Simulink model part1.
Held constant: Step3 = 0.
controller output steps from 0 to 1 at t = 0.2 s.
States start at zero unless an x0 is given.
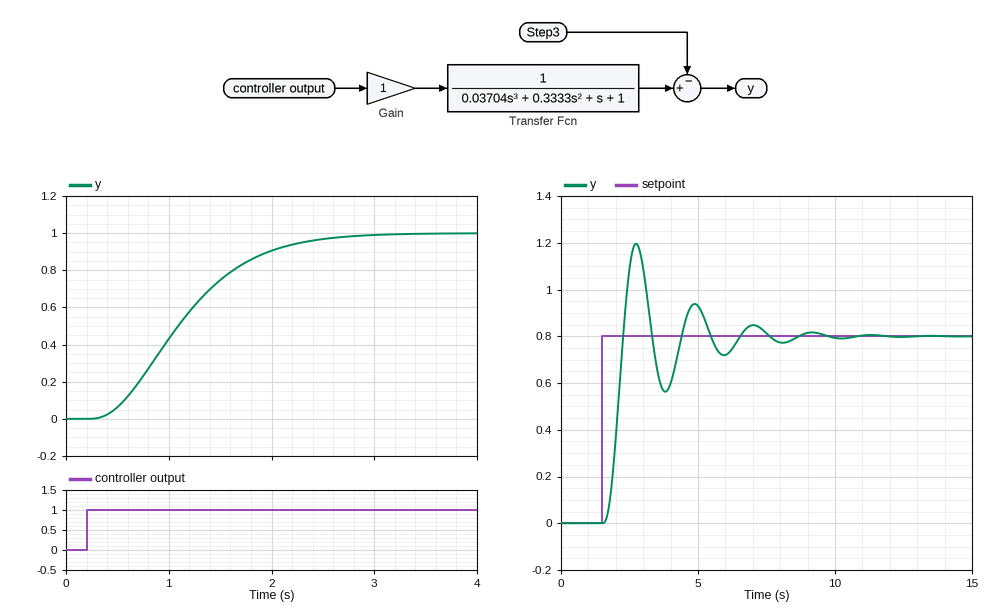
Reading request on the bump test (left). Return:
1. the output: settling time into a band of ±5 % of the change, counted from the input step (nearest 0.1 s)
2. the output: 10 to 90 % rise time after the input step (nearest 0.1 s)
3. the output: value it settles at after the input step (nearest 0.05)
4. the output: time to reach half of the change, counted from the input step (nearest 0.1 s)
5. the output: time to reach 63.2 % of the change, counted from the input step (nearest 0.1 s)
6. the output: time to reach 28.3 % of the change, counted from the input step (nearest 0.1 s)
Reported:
2.1 s
1.4 s
1.00
0.9 s
1.1 s
0.6 s
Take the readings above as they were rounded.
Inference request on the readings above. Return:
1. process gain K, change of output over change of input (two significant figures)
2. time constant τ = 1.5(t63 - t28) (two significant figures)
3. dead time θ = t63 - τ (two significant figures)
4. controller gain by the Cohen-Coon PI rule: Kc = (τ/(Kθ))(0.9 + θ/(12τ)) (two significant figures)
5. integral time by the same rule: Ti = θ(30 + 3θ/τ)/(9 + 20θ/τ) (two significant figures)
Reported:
1.0
0.75 s
0.35 s
2.0
0.60 s
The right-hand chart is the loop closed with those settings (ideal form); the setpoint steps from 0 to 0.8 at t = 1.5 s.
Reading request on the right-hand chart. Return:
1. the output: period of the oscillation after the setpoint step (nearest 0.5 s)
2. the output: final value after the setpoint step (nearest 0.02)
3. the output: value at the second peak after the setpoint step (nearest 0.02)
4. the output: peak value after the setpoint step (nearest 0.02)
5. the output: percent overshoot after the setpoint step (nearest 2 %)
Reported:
2.0 s
0.80
0.94
1.20
50 %
